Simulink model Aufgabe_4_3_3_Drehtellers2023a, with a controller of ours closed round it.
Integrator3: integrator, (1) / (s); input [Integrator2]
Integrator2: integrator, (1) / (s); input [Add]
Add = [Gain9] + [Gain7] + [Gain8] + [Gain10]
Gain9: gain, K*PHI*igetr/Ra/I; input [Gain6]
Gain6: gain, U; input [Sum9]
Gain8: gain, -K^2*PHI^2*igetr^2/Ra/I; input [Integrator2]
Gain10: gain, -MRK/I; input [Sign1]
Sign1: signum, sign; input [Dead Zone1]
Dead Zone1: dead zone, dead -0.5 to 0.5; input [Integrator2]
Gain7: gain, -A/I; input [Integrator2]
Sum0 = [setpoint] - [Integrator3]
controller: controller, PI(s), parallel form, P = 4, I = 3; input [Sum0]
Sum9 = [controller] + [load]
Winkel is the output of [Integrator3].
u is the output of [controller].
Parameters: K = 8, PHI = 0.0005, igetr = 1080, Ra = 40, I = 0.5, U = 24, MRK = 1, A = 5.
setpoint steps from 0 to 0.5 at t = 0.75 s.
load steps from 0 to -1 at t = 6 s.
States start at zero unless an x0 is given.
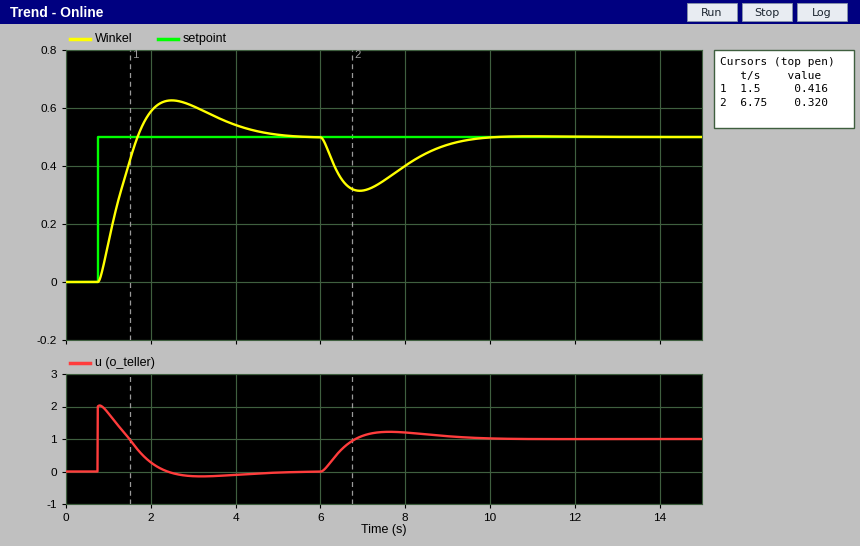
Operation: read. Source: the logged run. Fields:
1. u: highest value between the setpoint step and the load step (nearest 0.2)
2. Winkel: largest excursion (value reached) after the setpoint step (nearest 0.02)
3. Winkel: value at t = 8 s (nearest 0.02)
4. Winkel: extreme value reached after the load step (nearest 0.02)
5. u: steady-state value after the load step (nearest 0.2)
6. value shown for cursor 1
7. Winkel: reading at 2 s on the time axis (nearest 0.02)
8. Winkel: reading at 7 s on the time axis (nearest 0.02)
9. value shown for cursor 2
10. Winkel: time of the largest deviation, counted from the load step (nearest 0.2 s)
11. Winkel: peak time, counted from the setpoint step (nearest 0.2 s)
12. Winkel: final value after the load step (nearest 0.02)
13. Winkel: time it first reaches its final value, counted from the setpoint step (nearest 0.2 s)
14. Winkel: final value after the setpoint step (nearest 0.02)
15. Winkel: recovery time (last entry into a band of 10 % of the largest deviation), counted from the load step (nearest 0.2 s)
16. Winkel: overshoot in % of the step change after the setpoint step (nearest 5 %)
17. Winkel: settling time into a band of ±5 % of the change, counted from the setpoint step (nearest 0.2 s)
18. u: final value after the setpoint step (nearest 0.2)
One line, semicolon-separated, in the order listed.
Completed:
2.0; 0.62; 0.40; 0.32; 1.0; 0.416; 0.58; 0.32; 0.320; 1.0 s; 1.8 s; 0.50; 1.0 s; 0.50; 3.2 s; 25 %; 3.6 s; 0.0
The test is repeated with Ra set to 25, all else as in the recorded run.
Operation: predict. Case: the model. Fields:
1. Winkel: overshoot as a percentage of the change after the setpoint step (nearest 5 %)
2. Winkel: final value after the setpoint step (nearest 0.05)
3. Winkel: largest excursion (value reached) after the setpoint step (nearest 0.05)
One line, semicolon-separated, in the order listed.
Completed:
20 %; 0.50; 0.60
